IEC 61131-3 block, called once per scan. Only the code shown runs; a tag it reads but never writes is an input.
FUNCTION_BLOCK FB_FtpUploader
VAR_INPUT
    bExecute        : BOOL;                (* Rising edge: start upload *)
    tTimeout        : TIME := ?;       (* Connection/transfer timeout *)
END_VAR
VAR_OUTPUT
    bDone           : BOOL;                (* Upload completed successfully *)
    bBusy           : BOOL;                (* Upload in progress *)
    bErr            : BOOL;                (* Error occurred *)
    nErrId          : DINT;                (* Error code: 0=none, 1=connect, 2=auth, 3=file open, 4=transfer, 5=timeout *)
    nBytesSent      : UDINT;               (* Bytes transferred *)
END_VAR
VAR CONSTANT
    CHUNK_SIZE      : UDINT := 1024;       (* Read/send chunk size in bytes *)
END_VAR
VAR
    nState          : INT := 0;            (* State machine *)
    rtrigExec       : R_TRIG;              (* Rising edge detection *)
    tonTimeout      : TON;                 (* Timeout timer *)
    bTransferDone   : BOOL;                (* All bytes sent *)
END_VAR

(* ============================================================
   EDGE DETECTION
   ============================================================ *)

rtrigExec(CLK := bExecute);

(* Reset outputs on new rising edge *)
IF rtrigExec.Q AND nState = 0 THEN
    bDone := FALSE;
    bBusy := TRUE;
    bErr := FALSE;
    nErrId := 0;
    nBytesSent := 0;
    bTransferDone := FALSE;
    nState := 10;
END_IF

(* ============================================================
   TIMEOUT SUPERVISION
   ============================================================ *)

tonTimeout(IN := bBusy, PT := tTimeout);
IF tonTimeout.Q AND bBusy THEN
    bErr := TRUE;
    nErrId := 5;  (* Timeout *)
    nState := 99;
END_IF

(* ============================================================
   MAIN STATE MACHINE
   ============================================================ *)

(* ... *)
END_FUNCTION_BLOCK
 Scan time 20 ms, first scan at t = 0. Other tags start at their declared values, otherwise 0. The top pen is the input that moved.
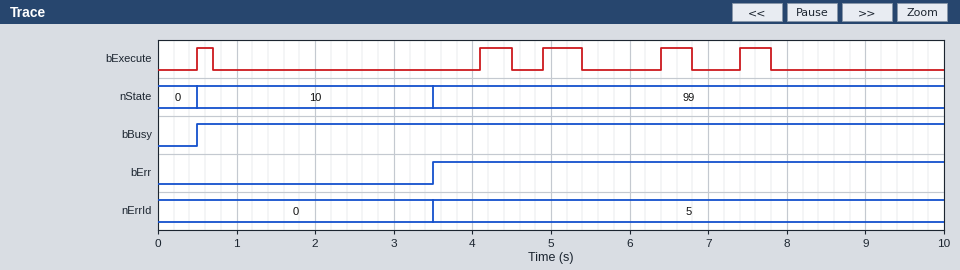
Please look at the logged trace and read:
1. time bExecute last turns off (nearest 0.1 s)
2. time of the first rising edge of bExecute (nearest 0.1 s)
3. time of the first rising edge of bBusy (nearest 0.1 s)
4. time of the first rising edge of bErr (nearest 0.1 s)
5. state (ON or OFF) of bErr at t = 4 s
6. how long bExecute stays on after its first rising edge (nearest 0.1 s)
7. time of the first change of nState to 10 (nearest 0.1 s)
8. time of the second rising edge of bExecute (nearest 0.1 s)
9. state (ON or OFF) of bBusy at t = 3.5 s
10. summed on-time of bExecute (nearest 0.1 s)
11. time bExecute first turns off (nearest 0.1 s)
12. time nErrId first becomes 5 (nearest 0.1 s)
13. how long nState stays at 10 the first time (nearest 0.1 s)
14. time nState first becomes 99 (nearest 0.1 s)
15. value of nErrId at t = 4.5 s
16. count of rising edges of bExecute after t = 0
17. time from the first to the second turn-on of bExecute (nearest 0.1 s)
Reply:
7.8 s
0.5 s
0.5 s
3.5 s
ON
0.2 s
0.5 s
4.1 s
ON
1.9 s
0.7 s
3.5 s
3.0 s
3.5 s
5
5
3.6 s
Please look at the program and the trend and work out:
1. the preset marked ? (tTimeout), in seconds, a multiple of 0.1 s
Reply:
3.0 s
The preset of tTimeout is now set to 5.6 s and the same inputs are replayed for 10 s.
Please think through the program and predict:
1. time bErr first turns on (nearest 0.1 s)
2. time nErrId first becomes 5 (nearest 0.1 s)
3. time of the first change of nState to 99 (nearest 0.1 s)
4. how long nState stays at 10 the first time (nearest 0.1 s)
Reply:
6.1 s
6.1 s
6.1 s
5.6 s
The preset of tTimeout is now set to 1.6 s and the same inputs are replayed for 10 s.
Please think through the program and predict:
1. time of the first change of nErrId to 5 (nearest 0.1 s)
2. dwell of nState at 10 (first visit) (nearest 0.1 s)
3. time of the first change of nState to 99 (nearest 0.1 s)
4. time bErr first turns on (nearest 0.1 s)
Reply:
2.1 s
1.6 s
2.1 s
2.1 s
